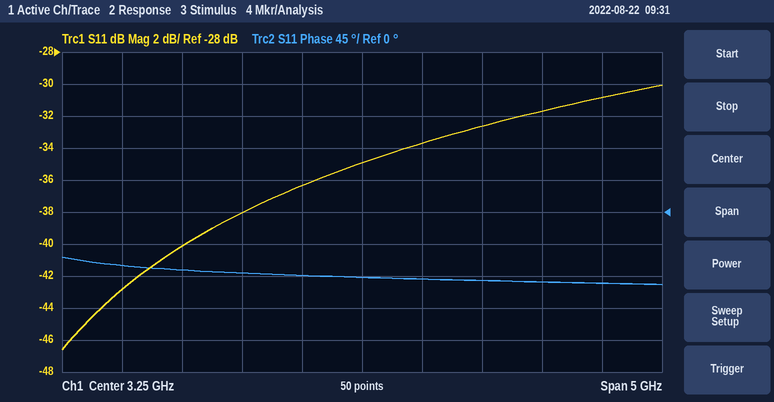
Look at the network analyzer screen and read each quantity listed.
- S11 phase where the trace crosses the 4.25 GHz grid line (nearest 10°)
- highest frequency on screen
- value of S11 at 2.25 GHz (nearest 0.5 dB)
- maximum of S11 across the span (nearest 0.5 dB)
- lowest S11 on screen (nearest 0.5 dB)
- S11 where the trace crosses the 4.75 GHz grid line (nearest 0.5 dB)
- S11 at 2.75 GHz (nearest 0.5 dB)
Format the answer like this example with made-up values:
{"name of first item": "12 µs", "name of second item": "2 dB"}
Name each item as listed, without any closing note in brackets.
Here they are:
{"S11 phase where the trace crosses the 4.25 GHz grid line": "-100°", "highest frequency on screen": "5.75 GHz", "value of S11 at 2.25 GHz": "-38.0 dB", "maximum of S11 across the span": "-30.0 dB", "lowest S11 on screen": "-46.5 dB", "S11 where the trace crosses the 4.75 GHz grid line": "-31.5 dB", "S11 at 2.75 GHz": "-36.5 dB"}
